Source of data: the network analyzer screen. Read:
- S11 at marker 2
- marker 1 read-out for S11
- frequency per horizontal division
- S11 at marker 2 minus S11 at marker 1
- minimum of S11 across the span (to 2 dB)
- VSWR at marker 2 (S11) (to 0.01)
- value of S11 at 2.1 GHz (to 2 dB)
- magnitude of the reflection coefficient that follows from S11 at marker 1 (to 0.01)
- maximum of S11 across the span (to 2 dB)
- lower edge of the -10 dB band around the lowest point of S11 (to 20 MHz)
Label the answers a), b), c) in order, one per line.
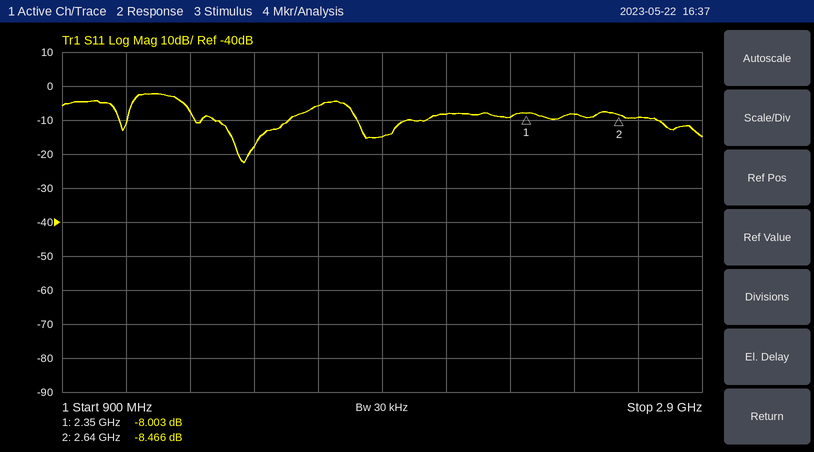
a) -8.466 dB
b) -8.003 dB
c) 200 MHz
d) -0.463 dB
e) -22 dB
f) 2.21
g) -8 dB
h) 0.40
i) -2 dB
j) 1.38 GHz
